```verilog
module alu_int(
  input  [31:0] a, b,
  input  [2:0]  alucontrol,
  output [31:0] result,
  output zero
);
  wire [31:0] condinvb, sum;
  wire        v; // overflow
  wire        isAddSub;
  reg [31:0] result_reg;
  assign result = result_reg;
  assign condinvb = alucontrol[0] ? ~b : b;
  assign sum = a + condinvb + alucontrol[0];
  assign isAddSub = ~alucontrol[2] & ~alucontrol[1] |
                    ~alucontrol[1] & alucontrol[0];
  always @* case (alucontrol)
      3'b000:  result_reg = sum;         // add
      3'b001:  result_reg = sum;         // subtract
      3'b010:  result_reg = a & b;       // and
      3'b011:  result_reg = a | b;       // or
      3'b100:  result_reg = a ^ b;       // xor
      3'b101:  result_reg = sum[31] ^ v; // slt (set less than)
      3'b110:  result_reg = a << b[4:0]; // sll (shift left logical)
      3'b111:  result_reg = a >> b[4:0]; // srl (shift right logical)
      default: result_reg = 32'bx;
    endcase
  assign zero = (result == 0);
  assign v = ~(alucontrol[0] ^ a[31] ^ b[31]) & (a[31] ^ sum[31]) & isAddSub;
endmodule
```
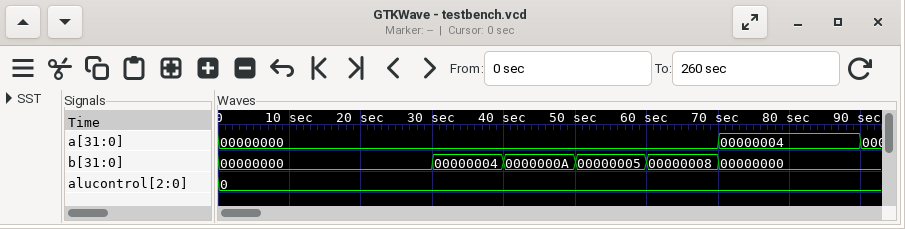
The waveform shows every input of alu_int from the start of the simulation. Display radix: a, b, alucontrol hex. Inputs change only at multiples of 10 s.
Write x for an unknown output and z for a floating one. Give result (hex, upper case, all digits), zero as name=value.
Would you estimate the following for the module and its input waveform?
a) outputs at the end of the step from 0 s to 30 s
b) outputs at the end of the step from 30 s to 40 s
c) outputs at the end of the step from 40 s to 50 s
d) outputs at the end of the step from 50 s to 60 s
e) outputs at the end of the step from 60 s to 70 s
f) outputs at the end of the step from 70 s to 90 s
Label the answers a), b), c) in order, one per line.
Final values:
a) result=00000000, zero=1
b) result=00000004, zero=0
c) result=0000000A, zero=0
d) result=00000005, zero=0
e) result=00000008, zero=0
f) result=00000004, zero=0
